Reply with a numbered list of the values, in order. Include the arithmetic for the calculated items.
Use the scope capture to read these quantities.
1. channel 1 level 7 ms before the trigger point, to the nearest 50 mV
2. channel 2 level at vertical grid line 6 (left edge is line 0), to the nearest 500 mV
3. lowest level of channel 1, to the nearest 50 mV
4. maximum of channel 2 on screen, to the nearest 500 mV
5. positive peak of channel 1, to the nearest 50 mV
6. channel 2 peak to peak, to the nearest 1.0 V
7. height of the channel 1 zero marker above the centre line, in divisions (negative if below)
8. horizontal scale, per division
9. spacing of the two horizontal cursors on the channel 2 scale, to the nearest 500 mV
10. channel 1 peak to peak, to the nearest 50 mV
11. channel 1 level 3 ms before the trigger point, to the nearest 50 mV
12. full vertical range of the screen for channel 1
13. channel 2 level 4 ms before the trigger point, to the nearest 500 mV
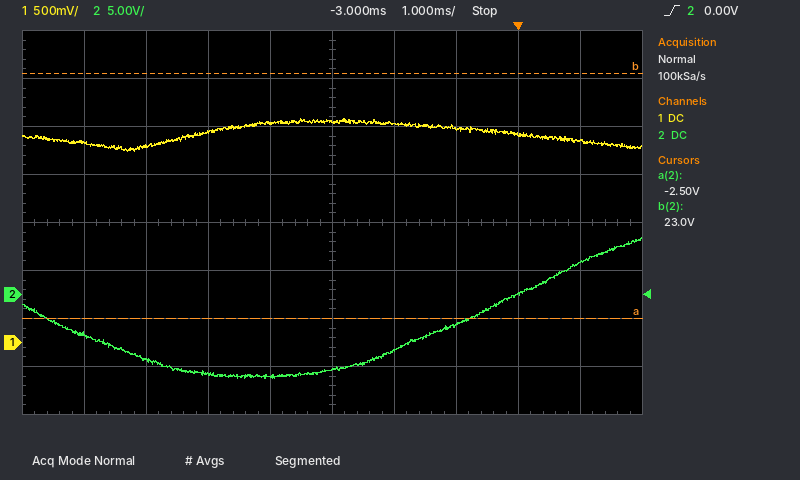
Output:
1. 2.10 V
2. -6.0 V
3. 2.00 V
4. 6.0 V
5. 2.35 V
6. 15.0 V
7. -2.5 div
8. 1 ms
9. 25.5 V
10. 2.35 V − (2.00 V) = 350 mV
11. 2.30 V
12. 4 V
13. -8.5 V
